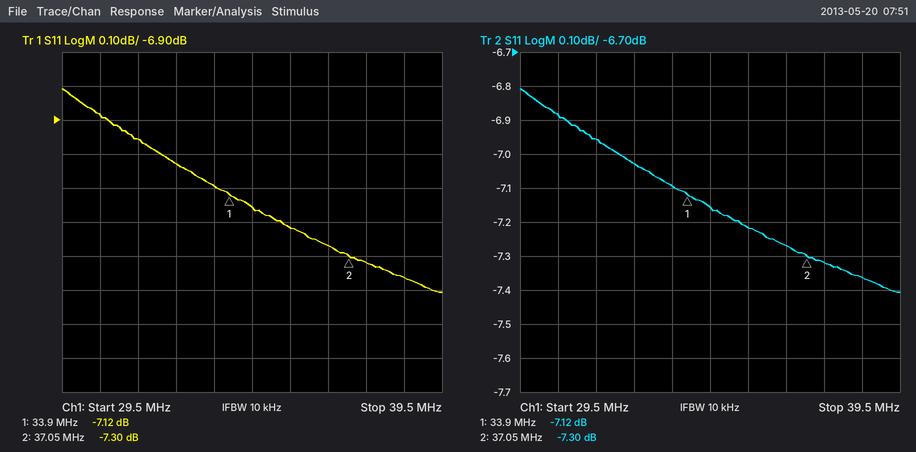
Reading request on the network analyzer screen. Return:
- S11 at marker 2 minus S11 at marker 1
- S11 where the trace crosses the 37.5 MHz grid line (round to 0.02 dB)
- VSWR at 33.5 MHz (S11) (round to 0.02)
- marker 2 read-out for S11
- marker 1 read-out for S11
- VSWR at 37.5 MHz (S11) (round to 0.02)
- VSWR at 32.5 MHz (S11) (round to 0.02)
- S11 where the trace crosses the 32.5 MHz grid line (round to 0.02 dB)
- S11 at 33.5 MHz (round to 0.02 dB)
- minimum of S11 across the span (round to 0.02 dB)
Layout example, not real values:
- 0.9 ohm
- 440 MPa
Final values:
- -0.18 dB
- -7.32 dB
- 2.58
- -7.30 dB
- -7.12 dB
- 2.52
- 2.60
- -7.02 dB
- -7.10 dB
- -7.40 dB
